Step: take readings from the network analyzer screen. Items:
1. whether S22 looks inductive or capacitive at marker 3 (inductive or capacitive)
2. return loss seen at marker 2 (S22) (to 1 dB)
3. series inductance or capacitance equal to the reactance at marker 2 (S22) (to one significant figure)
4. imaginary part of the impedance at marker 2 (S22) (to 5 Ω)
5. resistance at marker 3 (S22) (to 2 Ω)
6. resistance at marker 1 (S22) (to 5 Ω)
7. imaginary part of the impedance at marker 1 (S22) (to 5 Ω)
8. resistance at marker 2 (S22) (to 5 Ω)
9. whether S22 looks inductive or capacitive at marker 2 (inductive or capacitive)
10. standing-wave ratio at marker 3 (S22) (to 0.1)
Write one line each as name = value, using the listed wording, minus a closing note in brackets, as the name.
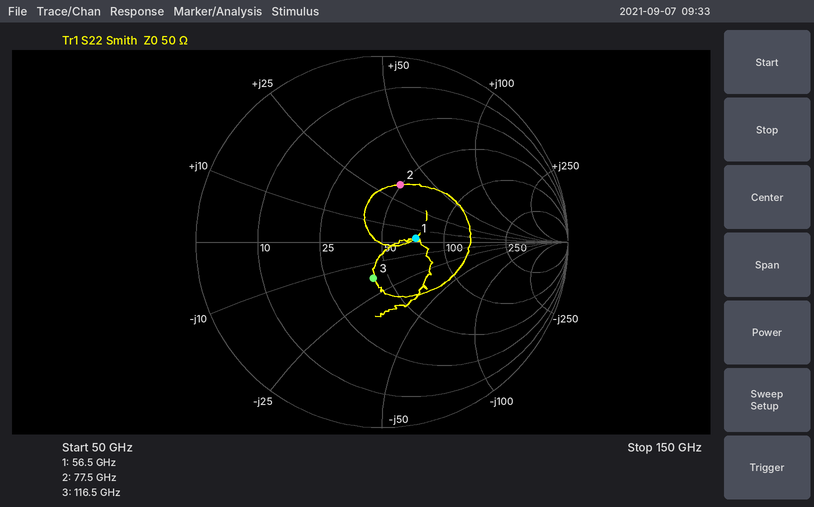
whether S22 looks inductive or capacitive at marker 3 = capacitive
return loss seen at marker 2 (S22) = 10 dB
series inductance or capacitance equal to the reactance at marker 2 (S22) = 70 pH
imaginary part of the impedance at marker 2 (S22) = +35 Ω
resistance at marker 3 (S22) = 42 Ω
resistance at marker 1 (S22) = 70 Ω
imaginary part of the impedance at marker 1 (S22) = +5 Ω
resistance at marker 2 (S22) = 50 Ω
whether S22 looks inductive or capacitive at marker 2 = inductive
standing-wave ratio at marker 3 (S22) = 1.5
